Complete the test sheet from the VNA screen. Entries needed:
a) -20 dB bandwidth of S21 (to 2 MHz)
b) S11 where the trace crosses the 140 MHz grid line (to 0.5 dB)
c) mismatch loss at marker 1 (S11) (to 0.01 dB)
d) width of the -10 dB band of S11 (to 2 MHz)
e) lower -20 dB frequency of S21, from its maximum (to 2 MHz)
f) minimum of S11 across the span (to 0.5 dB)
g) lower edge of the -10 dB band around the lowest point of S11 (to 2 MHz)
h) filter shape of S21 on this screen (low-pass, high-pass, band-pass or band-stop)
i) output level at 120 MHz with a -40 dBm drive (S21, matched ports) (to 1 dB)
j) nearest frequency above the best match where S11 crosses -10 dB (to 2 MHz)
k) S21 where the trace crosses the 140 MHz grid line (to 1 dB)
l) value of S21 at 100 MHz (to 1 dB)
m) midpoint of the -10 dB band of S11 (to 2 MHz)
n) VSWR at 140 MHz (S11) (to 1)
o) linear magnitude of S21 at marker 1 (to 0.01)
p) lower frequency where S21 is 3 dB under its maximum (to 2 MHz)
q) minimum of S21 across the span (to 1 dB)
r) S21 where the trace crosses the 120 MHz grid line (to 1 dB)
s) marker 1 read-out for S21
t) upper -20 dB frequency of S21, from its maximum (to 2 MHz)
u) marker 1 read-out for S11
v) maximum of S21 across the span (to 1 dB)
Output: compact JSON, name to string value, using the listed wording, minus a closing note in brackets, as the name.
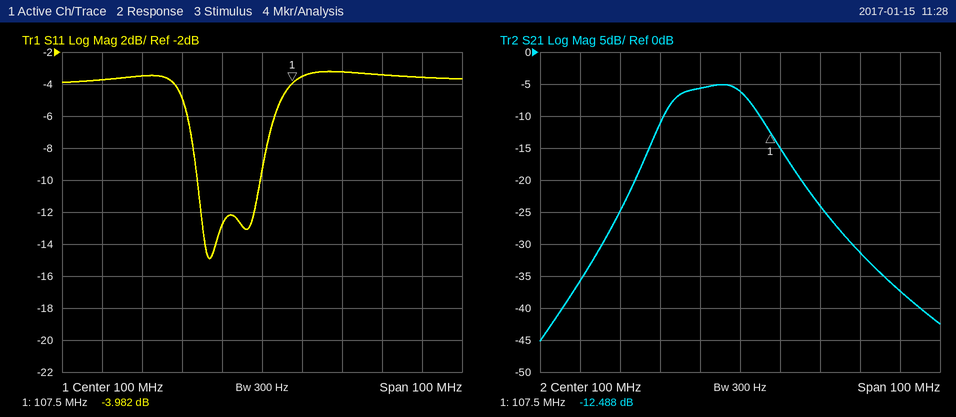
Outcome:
{"-20 dB bandwidth of S21": "52 MHz", "S11 where the trace crosses the 140 MHz grid line": "-3.5 dB", "mismatch loss at marker 1 (S11)": "2.22 dB", "width of the -10 dB band of S11": "16 MHz", "lower -20 dB frequency of S21, from its maximum": "70 MHz", "minimum of S11 across the span": "-15.0 dB", "lower edge of the -10 dB band around the lowest point of S11": "84 MHz", "filter shape of S21 on this screen": "band-pass", "output level at 120 MHz with a -40 dBm drive (S21, matched ports)": "-64 dBm", "nearest frequency above the best match where S11 crosses -10 dB": "100 MHz", "S21 where the trace crosses the 140 MHz grid line": "-37 dB", "value of S21 at 100 MHz": "-6 dB", "midpoint of the -10 dB band of S11": "92 MHz", "VSWR at 140 MHz (S11)": "5", "linear magnitude of S21 at marker 1": "0.24", "lower frequency where S21 is 3 dB under its maximum": "82 MHz", "minimum of S21 across the span": "-45 dB", "S21 where the trace crosses the 120 MHz grid line": "-24 dB", "marker 1 read-out for S21": "-12.488 dB", "upper -20 dB frequency of S21, from its maximum": "122 MHz", "marker 1 read-out for S11": "-3.982 dB", "maximum of S21 across the span": "-5 dB"}
